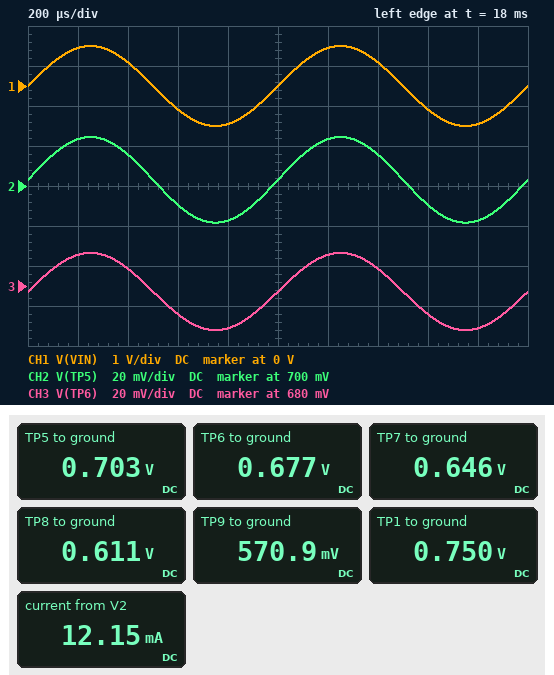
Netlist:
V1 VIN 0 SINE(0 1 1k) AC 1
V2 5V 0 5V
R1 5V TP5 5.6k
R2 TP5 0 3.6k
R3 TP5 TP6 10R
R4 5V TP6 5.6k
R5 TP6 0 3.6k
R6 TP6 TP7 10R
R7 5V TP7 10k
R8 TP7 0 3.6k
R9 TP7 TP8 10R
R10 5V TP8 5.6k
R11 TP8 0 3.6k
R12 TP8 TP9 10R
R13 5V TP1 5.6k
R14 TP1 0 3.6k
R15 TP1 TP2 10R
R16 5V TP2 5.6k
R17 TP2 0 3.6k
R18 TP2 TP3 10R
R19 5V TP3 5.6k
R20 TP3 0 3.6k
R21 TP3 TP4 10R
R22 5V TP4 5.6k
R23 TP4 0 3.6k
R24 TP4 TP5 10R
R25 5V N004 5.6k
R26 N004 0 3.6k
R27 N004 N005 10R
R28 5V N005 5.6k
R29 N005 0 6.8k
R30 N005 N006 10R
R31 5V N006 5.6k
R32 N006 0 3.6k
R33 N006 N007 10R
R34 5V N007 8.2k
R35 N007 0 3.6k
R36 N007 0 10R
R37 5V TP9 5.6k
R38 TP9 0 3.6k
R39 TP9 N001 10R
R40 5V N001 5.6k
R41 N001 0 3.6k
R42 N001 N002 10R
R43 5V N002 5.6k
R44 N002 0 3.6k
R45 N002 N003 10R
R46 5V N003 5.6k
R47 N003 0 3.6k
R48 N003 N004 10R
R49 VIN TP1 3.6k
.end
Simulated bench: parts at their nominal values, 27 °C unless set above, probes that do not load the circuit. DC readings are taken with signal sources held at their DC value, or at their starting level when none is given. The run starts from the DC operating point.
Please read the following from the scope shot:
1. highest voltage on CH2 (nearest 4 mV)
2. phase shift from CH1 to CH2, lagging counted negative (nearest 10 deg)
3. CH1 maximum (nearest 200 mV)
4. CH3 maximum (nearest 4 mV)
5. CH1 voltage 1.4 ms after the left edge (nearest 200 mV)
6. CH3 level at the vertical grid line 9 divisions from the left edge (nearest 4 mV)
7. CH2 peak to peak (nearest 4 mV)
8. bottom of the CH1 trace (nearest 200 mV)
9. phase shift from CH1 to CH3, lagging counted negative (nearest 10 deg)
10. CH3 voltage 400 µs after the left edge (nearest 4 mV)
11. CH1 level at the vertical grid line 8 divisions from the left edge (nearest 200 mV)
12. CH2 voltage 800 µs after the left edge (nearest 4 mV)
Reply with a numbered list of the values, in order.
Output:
1. 724 mV
2. 0 deg
3. 1.0 V
4. 696 mV
5. 600 mV
6. 660 mV
7. 44 mV
8. -1.0 V
9. 0 deg
10. 688 mV
11. -600 mV
12. 684 mV
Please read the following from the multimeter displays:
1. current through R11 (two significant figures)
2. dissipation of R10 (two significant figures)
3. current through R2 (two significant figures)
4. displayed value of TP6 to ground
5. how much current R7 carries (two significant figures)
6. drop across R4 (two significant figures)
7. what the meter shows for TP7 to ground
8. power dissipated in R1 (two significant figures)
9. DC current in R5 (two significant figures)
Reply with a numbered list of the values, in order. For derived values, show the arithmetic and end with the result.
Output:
1. (611 mV) / 3.6 kΩ = 170 µA
2. (5 V - 611 mV)^2 / 5.6 kΩ = 3.4 mW
3. (703 mV) / 3.6 kΩ = 200 µA
4. 0.677 V
5. (5 V - 646 mV) / 10 kΩ = 440 µA
6. 5 V - 677 mV = 4.3 V
7. 0.646 V
8. (5 V - 703 mV)^2 / 5.6 kΩ = 3.3 mW
9. (677 mV) / 3.6 kΩ = 190 µA
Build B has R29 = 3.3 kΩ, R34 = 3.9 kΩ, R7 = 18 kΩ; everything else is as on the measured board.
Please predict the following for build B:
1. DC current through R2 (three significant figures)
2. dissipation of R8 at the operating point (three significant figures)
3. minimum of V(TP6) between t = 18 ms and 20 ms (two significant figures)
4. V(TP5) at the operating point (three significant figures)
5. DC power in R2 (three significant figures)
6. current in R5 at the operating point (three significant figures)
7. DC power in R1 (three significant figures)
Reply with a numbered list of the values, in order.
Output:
1. 193 µA
2. 112 µW
3. 650 mV
4. 694 mV
5. 134 µW
6. 185 µA
7. 3.31 mW
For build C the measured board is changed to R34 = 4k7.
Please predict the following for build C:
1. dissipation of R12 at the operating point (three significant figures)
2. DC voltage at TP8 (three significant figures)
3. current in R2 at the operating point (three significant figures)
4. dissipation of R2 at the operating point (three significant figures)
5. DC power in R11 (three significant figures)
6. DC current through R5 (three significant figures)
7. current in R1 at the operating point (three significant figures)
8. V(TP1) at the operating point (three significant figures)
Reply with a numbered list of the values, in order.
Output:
1. 162 µW
2. 614 mV
3. 196 µA
4. 138 µW
5. 105 µW
6. 189 µA
7. 767 µA
8. 753 mV
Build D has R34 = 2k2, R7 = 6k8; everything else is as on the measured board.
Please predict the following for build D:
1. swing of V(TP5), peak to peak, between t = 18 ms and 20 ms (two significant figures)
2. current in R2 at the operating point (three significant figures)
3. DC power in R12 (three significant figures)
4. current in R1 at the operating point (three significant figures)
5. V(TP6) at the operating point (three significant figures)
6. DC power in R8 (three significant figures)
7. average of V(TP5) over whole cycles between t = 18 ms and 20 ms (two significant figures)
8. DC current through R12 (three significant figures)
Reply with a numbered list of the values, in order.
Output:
1. 43 mV
2. 202 µA
3. 173 µW
4. 763 µA
5. 701 mV
6. 125 µW
7. 730 mV
8. 4.15 mA
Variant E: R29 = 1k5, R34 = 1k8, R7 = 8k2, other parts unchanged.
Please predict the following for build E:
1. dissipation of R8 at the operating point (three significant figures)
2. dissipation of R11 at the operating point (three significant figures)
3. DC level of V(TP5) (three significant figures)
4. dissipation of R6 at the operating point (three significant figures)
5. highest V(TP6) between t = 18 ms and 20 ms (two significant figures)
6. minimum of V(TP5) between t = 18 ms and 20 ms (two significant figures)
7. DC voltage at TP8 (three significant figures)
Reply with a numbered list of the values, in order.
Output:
1. 122 µW
2. 110 µW
3. 720 mV
4. 97.4 µW
5. 710 mV
6. 700 mV
7. 628 mV
